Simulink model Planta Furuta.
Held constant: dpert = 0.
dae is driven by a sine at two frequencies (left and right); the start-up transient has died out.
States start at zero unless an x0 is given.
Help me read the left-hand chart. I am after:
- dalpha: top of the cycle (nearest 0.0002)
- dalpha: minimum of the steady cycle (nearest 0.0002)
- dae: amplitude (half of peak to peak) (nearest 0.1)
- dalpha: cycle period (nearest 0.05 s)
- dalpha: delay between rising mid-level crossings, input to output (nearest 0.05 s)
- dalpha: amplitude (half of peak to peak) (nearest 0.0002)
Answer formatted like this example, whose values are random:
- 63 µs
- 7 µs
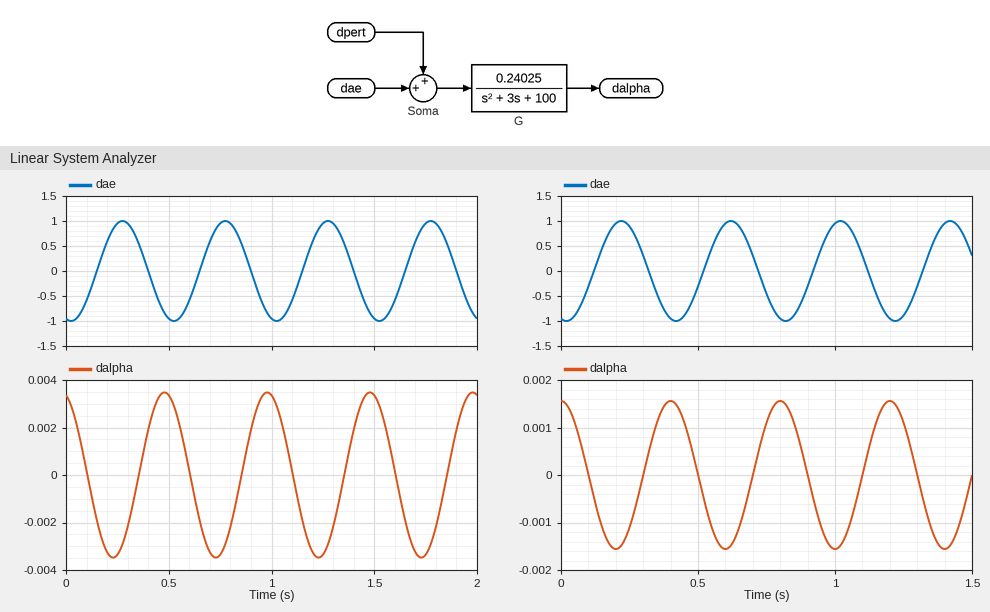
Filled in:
- 0.0034
- -0.0034
- 1.0
- 0.50 s
- 0.20 s
- 0.0034
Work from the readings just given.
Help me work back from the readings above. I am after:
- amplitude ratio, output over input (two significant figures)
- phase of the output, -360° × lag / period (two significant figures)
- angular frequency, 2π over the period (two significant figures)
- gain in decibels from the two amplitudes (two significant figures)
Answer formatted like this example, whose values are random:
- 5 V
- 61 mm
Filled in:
- 0.0034
- -140°
- 13 rad/s
- -49 dB
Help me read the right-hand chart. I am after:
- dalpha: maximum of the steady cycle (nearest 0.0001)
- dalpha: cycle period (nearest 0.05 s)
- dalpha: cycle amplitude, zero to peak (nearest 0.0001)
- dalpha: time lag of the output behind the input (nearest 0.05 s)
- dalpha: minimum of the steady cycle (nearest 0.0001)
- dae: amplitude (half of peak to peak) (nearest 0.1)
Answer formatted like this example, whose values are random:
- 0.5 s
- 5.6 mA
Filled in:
- 0.0016
- 0.40 s
- 0.0016
- 0.20 s
- -0.0016
- 1.0
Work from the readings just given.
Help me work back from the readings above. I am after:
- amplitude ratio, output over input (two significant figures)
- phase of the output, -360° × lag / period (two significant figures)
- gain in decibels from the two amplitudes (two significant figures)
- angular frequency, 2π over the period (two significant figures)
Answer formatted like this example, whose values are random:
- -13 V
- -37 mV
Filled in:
- 0.0016
- -180°
- -56 dB
- 16 rad/s
